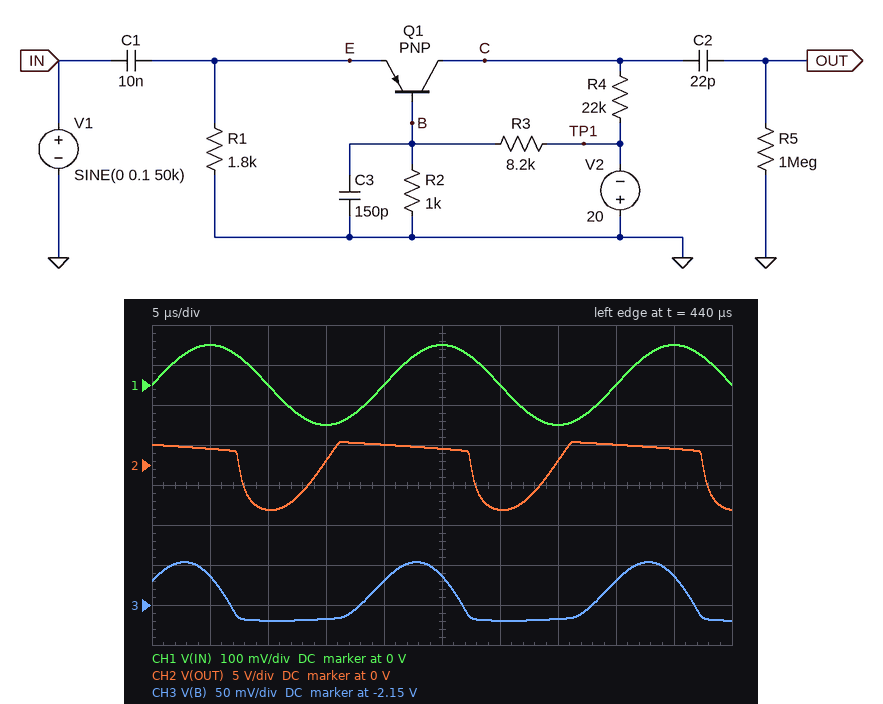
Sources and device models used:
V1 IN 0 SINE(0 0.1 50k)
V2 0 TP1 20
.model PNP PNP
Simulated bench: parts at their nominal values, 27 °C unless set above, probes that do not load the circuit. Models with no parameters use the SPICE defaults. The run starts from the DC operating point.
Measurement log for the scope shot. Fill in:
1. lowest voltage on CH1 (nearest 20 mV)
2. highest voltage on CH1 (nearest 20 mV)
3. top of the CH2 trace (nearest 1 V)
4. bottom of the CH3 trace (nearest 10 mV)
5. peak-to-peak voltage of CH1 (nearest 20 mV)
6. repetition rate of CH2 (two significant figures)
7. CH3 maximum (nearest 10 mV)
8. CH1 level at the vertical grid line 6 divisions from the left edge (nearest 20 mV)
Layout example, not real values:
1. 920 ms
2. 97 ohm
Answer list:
1. -100 mV
2. 100 mV
3. 3 V
4. -2.17 V
5. 200 mV
6. 50 kHz
7. -2.10 V
8. 0 V
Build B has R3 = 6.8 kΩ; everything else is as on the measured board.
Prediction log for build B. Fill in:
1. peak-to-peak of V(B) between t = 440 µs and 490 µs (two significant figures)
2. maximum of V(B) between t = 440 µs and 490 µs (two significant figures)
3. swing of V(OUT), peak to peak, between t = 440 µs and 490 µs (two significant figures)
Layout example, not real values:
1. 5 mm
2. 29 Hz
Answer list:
1. 160 mV
2. -2.4 V
3. 240 mV
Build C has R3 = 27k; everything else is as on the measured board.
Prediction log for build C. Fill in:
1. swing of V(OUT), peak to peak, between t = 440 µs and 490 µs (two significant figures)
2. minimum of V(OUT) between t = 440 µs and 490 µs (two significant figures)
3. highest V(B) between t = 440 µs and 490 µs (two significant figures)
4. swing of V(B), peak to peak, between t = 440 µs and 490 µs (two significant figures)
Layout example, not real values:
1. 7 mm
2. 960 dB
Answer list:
1. 3.7 V
2. -940 mV
3. -710 mV
4. 1.6 mV
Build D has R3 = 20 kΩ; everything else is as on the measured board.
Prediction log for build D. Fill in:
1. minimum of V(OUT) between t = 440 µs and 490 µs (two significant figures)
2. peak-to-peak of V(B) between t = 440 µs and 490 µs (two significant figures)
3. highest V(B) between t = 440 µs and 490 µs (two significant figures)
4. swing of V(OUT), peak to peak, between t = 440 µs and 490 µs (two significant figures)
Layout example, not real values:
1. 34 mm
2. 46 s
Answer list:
1. -2.9 V
2. 3.8 mV
3. -950 mV
4. 8.7 V
